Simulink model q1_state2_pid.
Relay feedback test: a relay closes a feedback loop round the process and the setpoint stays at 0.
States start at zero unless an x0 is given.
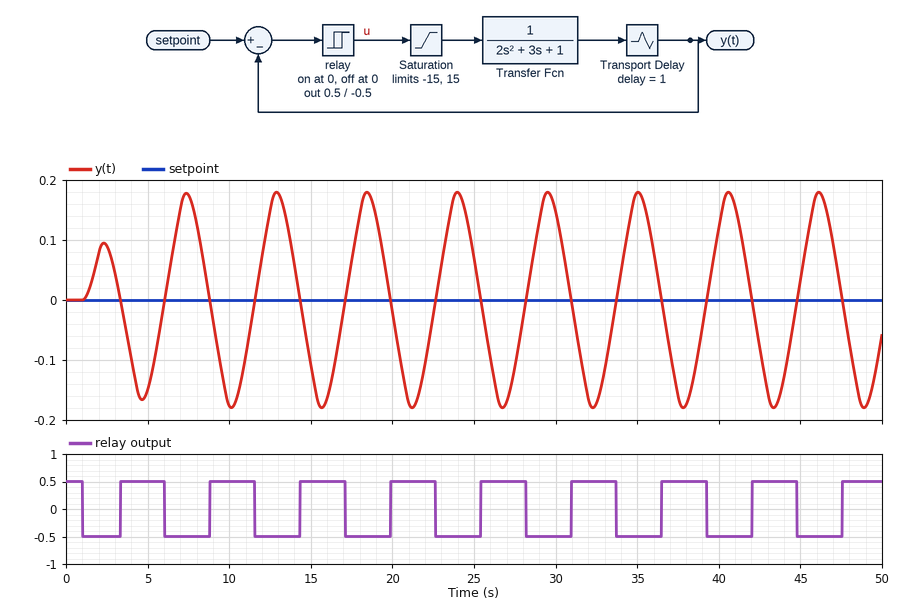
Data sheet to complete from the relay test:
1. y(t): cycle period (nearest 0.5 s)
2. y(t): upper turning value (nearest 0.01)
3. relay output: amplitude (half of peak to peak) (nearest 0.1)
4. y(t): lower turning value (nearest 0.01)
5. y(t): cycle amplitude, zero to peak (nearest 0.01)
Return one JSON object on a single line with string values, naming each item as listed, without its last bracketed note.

{"y(t): cycle period": "5.5 s", "y(t): upper turning value": "0.18", "relay output: amplitude (half of peak to peak)": "0.5", "y(t): lower turning value": "-0.18", "y(t): cycle amplitude, zero to peak": "0.18"}
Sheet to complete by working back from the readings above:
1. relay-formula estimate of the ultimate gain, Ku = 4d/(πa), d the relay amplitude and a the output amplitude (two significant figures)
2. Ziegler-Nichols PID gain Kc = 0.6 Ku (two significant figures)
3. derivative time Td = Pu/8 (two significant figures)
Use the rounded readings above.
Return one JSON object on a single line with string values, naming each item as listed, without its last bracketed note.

{"relay-formula estimate of the ultimate gain, Ku = 4d/(πa), d the relay amplitude and a the output amplitude": "3.5", "Ziegler-Nichols PID gain Kc = 0.6 Ku": "2.1", "derivative time Td = Pu/8": "0.69 s"}
